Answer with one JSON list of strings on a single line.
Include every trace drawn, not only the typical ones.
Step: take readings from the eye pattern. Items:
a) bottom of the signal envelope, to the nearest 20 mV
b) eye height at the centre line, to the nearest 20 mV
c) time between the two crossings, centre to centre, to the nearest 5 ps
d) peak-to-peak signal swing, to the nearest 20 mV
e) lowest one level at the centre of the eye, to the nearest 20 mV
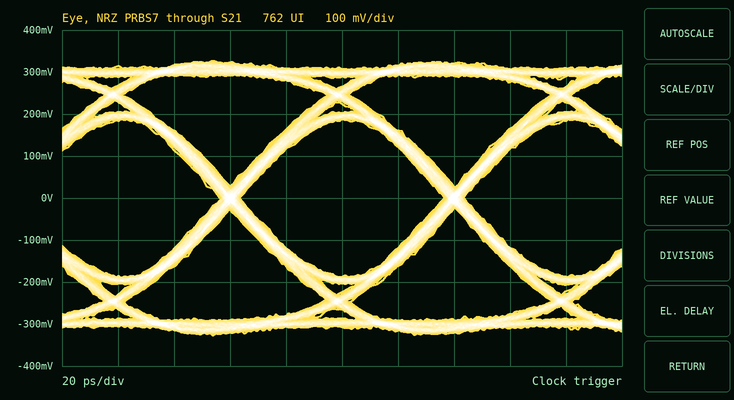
["-320 mV", "380 mV", "80 ps", "660 mV", "180 mV"]
